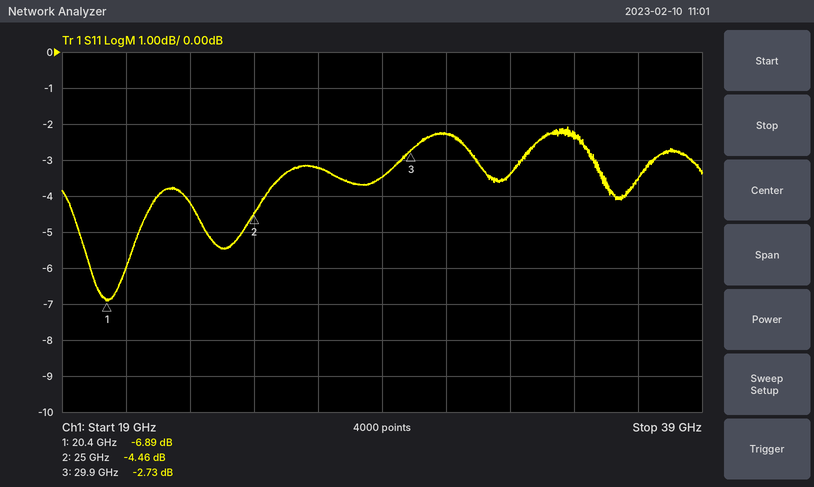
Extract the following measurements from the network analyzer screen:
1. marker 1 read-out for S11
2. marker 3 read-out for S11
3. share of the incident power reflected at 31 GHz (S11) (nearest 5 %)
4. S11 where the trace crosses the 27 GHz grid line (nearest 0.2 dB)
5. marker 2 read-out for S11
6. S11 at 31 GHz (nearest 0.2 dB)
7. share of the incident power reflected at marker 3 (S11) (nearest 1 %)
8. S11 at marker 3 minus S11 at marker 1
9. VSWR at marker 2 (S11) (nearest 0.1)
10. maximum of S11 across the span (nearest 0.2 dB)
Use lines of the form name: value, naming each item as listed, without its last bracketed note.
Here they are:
marker 1 read-out for S11: -6.89 dB
marker 3 read-out for S11: -2.73 dB
share of the incident power reflected at 31 GHz (S11): 60 %
S11 where the trace crosses the 27 GHz grid line: -3.2 dB
marker 2 read-out for S11: -4.46 dB
S11 at 31 GHz: -2.2 dB
share of the incident power reflected at marker 3 (S11): 53 %
S11 at marker 3 minus S11 at marker 1: 4.16 dB
VSWR at marker 2 (S11): 4.0
maximum of S11 across the span: -2.0 dB
